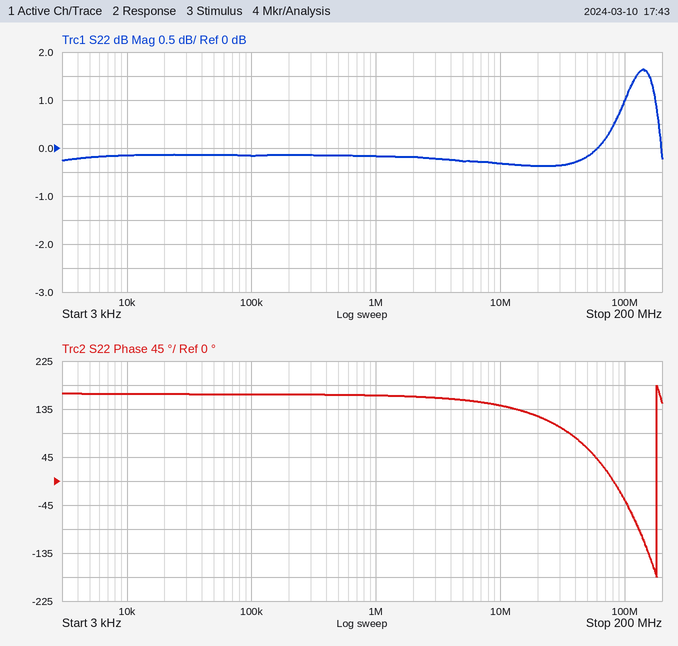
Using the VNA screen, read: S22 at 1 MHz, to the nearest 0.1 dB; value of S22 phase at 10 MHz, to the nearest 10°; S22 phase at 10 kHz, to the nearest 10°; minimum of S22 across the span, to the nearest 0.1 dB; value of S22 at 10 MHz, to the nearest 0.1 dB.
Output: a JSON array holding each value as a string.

["-0.2 dB", "140°", "160°", "-0.4 dB", "-0.3 dB"]
